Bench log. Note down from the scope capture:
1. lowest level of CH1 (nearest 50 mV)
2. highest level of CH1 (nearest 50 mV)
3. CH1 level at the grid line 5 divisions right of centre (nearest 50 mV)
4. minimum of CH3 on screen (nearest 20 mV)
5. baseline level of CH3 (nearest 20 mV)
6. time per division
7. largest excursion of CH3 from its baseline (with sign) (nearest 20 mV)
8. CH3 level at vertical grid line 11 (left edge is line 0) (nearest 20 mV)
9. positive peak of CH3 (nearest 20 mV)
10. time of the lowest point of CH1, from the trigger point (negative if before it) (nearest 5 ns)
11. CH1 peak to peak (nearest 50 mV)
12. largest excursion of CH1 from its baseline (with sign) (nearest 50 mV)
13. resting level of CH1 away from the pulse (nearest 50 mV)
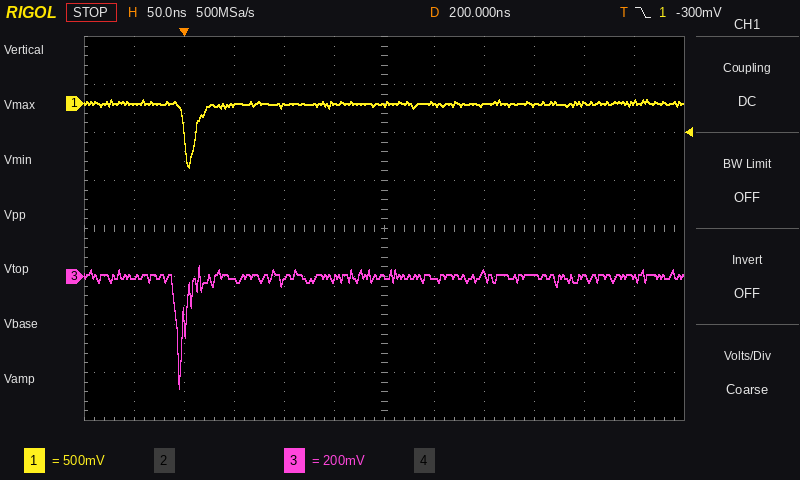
-650 mV
50 mV
0 mV
-460 mV
0 mV
50 ns
-460 mV
0 mV
40 mV
+5 ns
700 mV
-650 mV
0 mV
